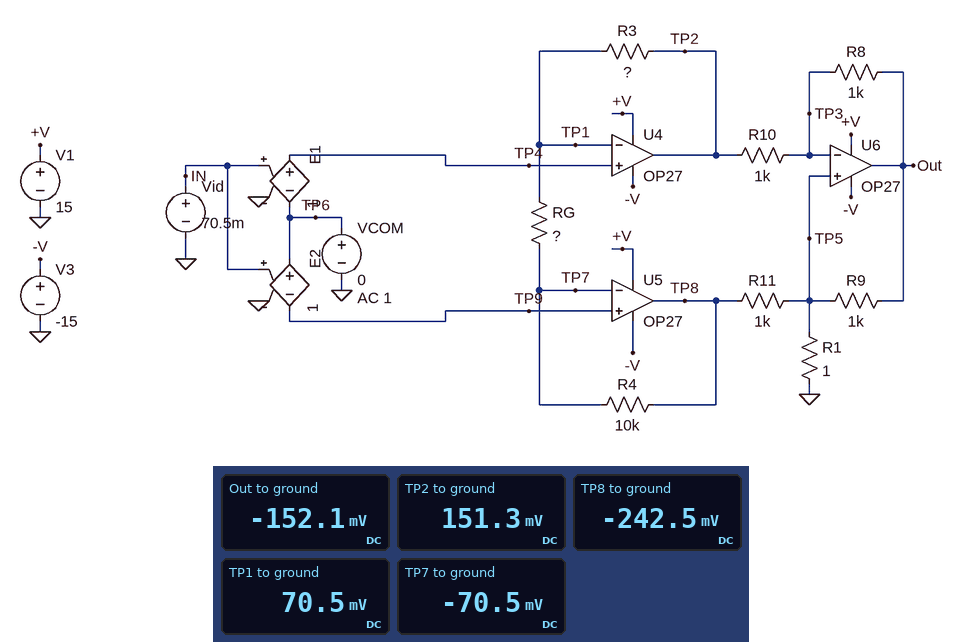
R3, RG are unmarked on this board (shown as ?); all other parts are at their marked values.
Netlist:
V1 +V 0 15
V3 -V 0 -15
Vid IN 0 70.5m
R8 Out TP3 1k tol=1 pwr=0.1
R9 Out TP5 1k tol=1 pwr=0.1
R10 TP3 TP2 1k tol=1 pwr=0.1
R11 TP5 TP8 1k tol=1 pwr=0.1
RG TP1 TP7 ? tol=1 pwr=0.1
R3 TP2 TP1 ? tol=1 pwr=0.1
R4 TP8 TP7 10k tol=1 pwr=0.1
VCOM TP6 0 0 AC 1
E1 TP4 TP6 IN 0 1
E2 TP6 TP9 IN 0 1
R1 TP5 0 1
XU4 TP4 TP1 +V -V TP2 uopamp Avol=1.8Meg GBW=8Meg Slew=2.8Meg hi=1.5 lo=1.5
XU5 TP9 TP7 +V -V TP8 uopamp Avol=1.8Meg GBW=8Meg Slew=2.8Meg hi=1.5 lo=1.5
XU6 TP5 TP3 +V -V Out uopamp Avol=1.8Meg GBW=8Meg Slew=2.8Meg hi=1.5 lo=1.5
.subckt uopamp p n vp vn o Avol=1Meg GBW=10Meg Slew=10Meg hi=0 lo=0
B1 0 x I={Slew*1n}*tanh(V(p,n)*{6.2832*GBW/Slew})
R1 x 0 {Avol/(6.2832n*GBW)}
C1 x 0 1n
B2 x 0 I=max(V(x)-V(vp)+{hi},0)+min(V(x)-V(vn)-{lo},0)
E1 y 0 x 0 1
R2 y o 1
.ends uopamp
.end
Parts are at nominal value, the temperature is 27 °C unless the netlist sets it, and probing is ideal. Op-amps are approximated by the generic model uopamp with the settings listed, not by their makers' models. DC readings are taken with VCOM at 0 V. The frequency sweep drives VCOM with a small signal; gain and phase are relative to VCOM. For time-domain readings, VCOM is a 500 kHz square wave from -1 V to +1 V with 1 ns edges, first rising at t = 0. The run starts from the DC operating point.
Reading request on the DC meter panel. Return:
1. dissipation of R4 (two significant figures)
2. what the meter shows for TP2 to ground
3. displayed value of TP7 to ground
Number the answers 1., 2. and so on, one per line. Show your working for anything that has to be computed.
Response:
1. (-70.5 mV - (-242.5 mV))^2 / 10 kΩ = 3.0 µW
2. 151.3 mV
3. -70.5 mV
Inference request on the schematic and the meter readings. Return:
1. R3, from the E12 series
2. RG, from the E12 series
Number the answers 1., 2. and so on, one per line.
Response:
1. 4.7 kΩ
2. 8.2 kΩ
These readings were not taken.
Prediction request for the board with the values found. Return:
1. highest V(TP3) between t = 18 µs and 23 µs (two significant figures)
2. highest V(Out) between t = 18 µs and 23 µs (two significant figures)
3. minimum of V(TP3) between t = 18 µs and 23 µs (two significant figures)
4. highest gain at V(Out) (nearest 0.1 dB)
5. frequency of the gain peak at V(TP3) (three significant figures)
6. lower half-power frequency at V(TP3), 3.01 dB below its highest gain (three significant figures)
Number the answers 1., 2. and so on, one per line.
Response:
1. 120 mV
2. 850 mV
3. -120 mV
4. 0 dB
5. 5.65 MHz
6. 2.24 MHz
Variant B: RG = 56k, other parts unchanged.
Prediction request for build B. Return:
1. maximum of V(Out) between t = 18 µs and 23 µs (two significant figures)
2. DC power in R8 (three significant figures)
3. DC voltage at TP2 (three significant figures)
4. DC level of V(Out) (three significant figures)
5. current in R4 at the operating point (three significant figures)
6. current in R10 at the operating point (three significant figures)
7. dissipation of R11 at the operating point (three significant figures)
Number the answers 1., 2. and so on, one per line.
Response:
1. 920 mV
2. 6.81 µW
3. 82.3 mV
4. -82.7 mV
5. 2.52 µA
6. 82.5 µA
7. 9.12 µW
